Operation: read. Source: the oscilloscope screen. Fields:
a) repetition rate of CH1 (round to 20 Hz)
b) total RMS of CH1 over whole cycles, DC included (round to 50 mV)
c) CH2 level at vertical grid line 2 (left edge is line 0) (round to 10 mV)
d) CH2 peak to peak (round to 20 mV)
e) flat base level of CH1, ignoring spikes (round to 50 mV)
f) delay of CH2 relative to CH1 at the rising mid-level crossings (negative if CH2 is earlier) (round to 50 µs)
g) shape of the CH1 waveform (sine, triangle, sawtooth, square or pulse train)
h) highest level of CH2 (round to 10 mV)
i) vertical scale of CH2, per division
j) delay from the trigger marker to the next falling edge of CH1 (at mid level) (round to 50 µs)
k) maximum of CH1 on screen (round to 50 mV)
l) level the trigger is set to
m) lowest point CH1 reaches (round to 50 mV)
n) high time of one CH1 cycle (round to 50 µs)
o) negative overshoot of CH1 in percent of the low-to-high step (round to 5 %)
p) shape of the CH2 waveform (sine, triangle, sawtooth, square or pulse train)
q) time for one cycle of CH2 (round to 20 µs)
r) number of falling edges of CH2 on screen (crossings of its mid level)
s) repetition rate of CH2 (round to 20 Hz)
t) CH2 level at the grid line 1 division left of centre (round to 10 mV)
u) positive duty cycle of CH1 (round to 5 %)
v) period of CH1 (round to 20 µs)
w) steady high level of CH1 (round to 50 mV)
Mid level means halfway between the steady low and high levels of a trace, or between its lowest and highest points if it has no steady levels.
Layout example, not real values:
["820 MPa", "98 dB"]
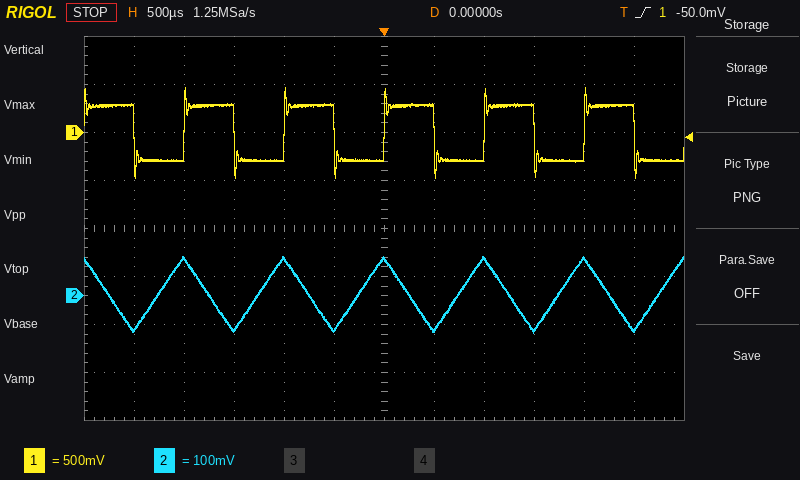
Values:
["1.00 kHz", "300 mV", "80 mV", "160 mV", "-300 mV", "-250 µs", "square", "80 mV", "100 mV", "500 µs", "450 mV", "-50.0 mV", "-450 mV", "500 µs", "30 %", "triangle", "1.00 ms", "6", "1.00 kHz", "-70 mV", "50 %", "1.00 ms", "300 mV"]
